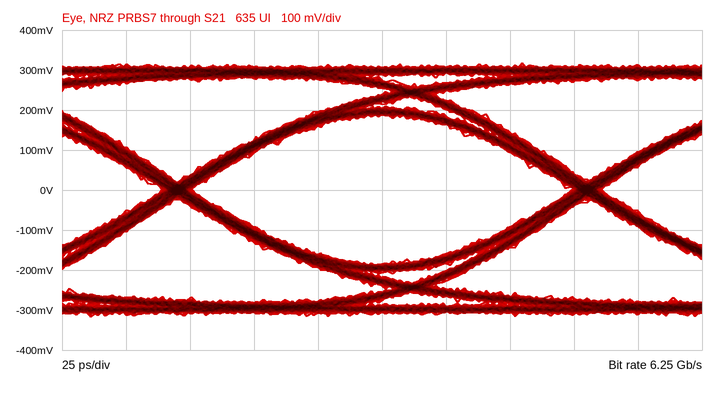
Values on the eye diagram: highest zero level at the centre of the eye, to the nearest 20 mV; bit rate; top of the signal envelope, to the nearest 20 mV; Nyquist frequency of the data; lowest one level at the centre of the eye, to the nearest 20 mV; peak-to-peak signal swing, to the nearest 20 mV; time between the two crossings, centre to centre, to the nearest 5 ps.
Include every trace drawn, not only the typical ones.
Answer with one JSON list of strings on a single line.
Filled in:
["-180 mV", "6.25 Gb/s", "320 mV", "3.125 GHz", "180 mV", "640 mV", "160 ps"]
